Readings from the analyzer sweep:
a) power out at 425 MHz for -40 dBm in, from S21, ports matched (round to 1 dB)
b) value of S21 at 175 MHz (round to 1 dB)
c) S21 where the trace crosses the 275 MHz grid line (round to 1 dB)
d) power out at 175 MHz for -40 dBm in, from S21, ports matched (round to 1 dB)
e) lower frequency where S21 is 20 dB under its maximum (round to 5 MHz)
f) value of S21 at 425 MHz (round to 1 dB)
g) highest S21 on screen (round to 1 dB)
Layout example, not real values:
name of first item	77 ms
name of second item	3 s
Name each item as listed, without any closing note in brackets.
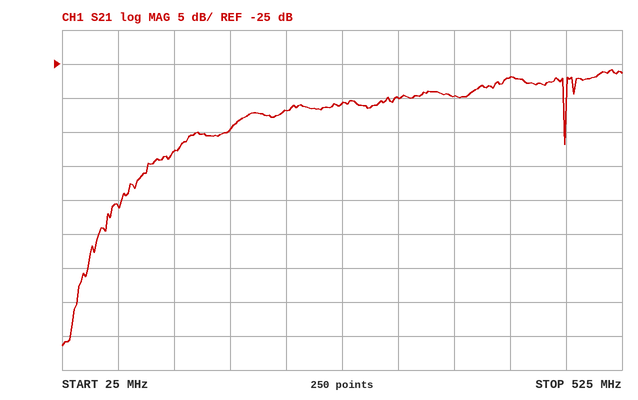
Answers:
power out at 425 MHz for -40 dBm in, from S21, ports matched	-67 dBm
value of S21 at 175 MHz	-35 dB
S21 where the trace crosses the 275 MHz grid line	-31 dB
power out at 175 MHz for -40 dBm in, from S21, ports matched	-75 dBm
lower frequency where S21 is 20 dB under its maximum	75 MHz
value of S21 at 425 MHz	-27 dB
highest S21 on screen	-26 dB
